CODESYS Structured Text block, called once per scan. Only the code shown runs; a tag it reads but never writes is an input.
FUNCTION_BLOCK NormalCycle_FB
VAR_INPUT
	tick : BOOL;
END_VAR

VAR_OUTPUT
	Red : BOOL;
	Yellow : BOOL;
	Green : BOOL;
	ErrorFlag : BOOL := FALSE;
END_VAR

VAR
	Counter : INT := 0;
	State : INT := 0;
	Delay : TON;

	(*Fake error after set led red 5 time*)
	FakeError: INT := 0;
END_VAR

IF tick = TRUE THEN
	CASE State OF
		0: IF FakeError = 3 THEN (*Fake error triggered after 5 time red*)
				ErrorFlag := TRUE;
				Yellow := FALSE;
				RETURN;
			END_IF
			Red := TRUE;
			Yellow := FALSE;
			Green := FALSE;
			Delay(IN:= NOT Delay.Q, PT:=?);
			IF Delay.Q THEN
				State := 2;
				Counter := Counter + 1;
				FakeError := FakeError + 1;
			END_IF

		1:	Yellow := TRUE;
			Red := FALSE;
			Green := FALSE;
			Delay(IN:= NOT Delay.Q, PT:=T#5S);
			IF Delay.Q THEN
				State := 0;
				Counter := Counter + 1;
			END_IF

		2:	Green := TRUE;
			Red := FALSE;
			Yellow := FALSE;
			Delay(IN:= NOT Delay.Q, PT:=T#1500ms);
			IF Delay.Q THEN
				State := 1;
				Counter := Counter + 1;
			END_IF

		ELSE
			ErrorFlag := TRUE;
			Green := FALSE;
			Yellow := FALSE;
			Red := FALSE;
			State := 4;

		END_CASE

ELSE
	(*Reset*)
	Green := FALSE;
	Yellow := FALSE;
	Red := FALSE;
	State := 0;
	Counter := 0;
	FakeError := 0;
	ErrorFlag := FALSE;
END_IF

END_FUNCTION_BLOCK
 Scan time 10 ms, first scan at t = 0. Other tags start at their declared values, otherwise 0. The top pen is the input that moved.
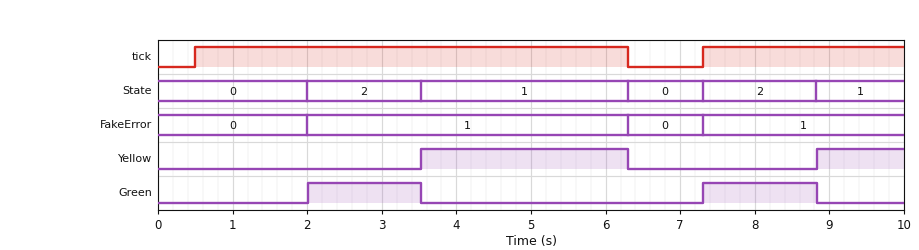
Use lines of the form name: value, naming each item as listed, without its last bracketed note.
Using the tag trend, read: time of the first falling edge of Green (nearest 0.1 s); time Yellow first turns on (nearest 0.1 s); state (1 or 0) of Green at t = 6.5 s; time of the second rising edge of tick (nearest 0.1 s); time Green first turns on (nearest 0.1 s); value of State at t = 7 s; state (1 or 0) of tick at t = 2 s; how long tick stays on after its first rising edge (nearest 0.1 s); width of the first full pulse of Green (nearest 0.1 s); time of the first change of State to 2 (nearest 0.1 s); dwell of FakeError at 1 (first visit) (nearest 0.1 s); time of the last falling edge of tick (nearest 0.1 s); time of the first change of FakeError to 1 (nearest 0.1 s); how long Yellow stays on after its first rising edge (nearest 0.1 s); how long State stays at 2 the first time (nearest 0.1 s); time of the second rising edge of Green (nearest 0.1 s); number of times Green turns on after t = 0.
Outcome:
time of the first falling edge of Green: 3.5 s
time Yellow first turns on: 3.5 s
state (1 or 0) of Green at t = 6.5 s: 0
time of the second rising edge of tick: 7.3 s
time Green first turns on: 2.0 s
value of State at t = 7 s: 0
state (1 or 0) of tick at t = 2 s: 1
how long tick stays on after its first rising edge: 5.8 s
width of the first full pulse of Green: 1.5 s
time of the first change of State to 2: 2.0 s
dwell of FakeError at 1 (first visit): 4.3 s
time of the last falling edge of tick: 6.3 s
time of the first change of FakeError to 1: 2.0 s
how long Yellow stays on after its first rising edge: 2.8 s
how long State stays at 2 the first time: 1.5 s
time of the second rising edge of Green: 7.3 s
number of times Green turns on after t = 0: 2
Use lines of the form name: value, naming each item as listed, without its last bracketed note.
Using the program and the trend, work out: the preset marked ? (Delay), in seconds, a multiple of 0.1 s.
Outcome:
the preset marked ? (Delay), in seconds, a multiple of 0.1 s: 1.5 s
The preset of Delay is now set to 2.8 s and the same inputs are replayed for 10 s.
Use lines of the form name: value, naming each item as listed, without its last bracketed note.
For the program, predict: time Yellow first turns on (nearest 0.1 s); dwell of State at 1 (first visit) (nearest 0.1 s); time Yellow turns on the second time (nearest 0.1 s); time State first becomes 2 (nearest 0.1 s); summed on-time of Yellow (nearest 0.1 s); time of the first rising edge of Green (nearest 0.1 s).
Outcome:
time Yellow first turns on: 4.8 s
dwell of State at 1 (first visit): 1.5 s
time Yellow turns on the second time: 9.2 s
time State first becomes 2: 3.3 s
summed on-time of Yellow: 2.3 s
time of the first rising edge of Green: 3.3 s
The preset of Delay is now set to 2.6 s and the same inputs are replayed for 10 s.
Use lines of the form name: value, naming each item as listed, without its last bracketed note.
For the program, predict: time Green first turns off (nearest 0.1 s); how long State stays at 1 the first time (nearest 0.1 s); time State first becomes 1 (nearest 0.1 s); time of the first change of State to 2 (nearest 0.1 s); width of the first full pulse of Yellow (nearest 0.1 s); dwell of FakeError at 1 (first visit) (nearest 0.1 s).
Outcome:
time Green first turns off: 4.6 s
how long State stays at 1 the first time: 1.7 s
time State first becomes 1: 4.6 s
time of the first change of State to 2: 3.1 s
width of the first full pulse of Yellow: 1.7 s
dwell of FakeError at 1 (first visit): 3.2 s
